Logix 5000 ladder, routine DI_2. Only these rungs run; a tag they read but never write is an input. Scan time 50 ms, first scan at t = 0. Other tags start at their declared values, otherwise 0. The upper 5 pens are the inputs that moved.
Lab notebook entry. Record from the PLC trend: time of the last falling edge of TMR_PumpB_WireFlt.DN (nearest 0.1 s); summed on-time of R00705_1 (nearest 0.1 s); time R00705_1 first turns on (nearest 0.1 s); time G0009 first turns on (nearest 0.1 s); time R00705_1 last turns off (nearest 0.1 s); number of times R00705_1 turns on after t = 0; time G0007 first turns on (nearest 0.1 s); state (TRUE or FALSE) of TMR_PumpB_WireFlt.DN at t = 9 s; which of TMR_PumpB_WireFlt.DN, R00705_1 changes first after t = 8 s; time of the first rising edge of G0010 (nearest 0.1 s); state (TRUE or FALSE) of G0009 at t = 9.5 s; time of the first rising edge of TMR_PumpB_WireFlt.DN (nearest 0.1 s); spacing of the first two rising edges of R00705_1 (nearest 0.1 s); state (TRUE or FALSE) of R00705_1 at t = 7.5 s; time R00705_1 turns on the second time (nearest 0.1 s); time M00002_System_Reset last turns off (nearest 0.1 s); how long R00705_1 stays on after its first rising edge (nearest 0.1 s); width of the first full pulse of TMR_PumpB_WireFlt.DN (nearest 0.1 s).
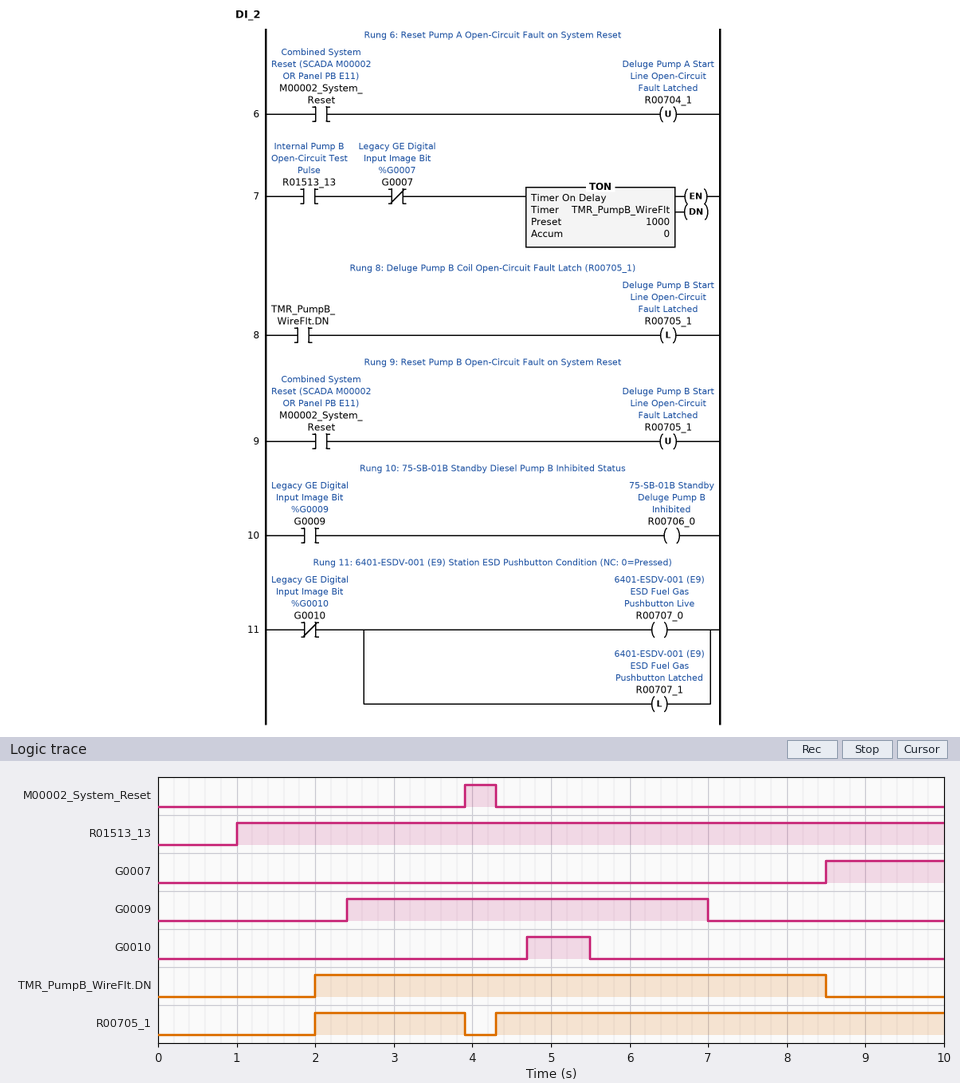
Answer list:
8.5 s
7.6 s
2.0 s
2.4 s
3.9 s
2
8.5 s
FALSE
TMR_PumpB_WireFlt.DN
4.7 s
FALSE
2.0 s
2.3 s
TRUE
4.3 s
4.3 s
1.9 s
6.5 s
